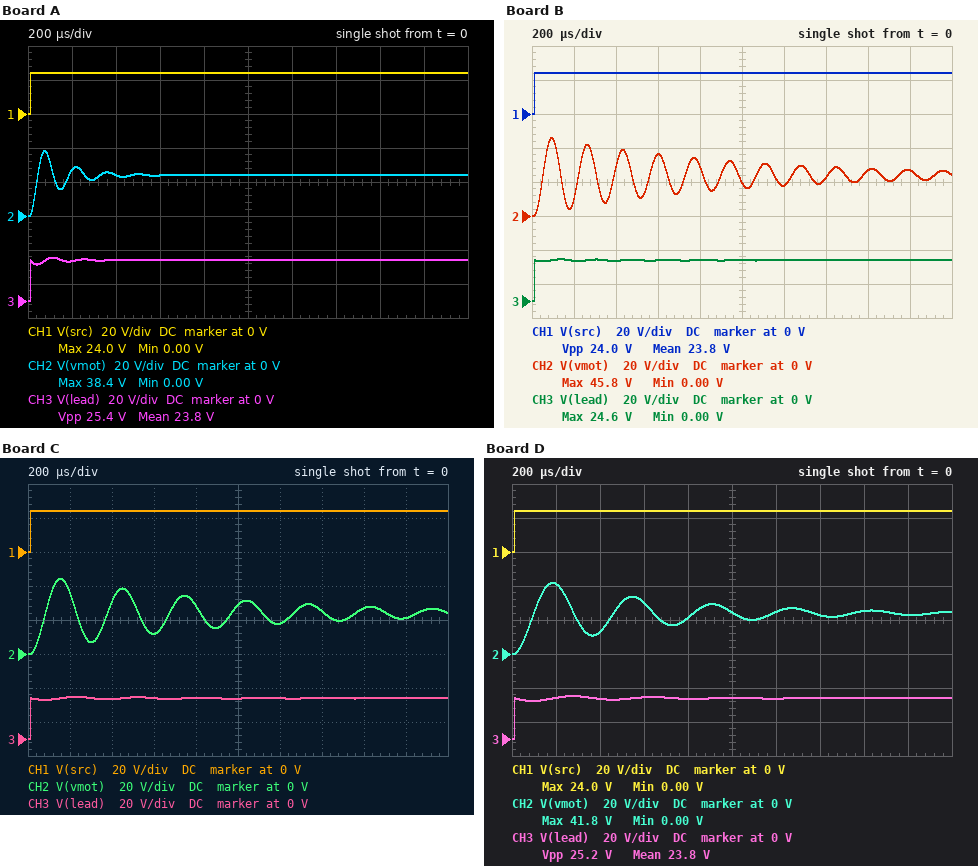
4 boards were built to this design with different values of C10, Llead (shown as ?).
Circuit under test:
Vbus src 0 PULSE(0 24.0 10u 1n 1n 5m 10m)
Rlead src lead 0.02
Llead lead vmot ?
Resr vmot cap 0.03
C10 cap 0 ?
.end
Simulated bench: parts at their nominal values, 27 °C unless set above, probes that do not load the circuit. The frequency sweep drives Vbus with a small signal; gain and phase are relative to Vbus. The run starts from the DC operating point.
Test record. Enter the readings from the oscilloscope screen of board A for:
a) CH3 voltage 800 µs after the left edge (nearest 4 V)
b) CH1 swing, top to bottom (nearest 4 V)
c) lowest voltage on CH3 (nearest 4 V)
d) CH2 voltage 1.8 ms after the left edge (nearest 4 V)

24 V
24 V
0 V
24 V
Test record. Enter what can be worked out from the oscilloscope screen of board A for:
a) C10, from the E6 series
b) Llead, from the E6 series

150 µF
3.3 µH
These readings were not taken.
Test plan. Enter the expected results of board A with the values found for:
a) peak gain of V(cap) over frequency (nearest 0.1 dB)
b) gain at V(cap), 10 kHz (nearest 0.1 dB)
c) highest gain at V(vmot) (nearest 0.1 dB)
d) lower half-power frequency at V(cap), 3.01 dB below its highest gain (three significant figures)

9.6 dB
-0.5 dB
9.7 dB
5.59 kHz
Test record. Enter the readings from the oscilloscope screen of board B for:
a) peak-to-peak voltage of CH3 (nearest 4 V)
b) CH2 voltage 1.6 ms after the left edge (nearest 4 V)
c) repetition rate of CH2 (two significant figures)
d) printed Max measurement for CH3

24 V
28 V
5.9 kHz
24.6 V
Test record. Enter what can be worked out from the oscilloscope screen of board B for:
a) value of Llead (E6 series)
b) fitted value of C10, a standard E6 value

22 µH
33 µF
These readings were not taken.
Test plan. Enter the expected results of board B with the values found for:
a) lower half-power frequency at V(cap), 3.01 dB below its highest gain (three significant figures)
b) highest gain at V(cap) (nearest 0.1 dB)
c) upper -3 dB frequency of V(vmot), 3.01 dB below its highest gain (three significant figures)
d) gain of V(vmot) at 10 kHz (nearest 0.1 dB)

5.72 kHz
24.3 dB
6.08 kHz
-5.4 dB
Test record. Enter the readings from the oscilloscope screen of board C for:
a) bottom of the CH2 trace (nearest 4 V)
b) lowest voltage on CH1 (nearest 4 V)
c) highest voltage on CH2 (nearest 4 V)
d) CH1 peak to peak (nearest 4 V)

0 V
0 V
44 V
24 V
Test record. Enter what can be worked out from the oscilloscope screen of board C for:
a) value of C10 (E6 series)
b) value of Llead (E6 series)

100 µF
22 µH
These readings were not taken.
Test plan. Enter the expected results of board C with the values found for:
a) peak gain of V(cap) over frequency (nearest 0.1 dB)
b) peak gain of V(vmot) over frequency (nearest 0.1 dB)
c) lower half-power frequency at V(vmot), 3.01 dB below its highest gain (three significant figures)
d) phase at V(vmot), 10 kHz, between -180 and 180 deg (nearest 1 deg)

19.5 dB
19.5 dB
3.20 kHz
-167 deg
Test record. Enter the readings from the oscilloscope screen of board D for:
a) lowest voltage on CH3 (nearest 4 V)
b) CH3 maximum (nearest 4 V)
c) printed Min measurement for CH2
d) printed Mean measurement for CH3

0 V
24 V
0.00 V
23.8 V
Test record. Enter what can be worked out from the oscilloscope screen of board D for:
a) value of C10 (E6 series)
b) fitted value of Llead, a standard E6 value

220 µF
15 µH
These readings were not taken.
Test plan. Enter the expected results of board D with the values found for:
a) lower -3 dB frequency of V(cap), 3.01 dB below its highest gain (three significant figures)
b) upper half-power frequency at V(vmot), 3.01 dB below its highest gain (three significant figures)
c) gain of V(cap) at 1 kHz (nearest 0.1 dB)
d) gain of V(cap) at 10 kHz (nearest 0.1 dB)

2.46 kHz
3.00 kHz
1.2 dB
-21.6 dB
